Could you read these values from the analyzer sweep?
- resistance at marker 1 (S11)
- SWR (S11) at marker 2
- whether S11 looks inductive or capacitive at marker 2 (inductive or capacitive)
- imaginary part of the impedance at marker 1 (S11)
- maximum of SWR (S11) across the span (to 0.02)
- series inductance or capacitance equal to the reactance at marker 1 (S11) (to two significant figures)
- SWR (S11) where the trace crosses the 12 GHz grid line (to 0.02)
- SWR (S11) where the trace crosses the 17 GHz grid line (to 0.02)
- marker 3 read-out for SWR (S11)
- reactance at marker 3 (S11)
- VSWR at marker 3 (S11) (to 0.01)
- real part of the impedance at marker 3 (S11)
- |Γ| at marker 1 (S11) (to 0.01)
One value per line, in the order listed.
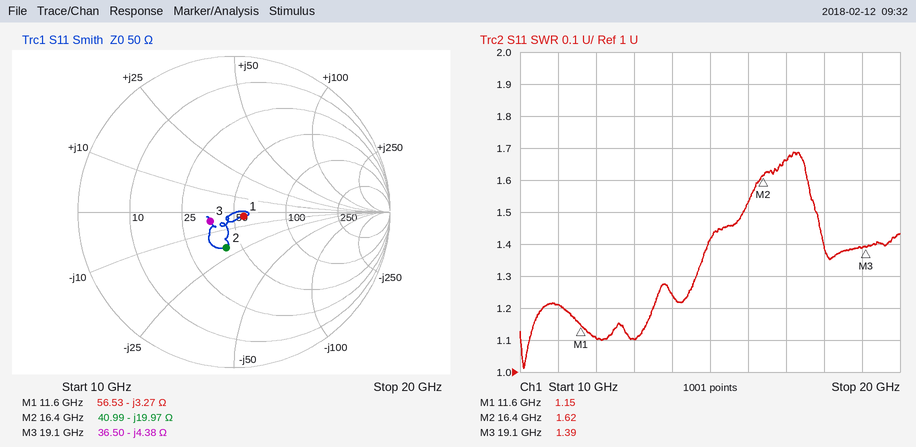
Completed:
56.53 Ω
1.62
capacitive
-3.27 Ω
1.68
4.2 pF
1.10
1.66
1.39
-4.38 Ω
1.39
36.50 Ω
0.07
